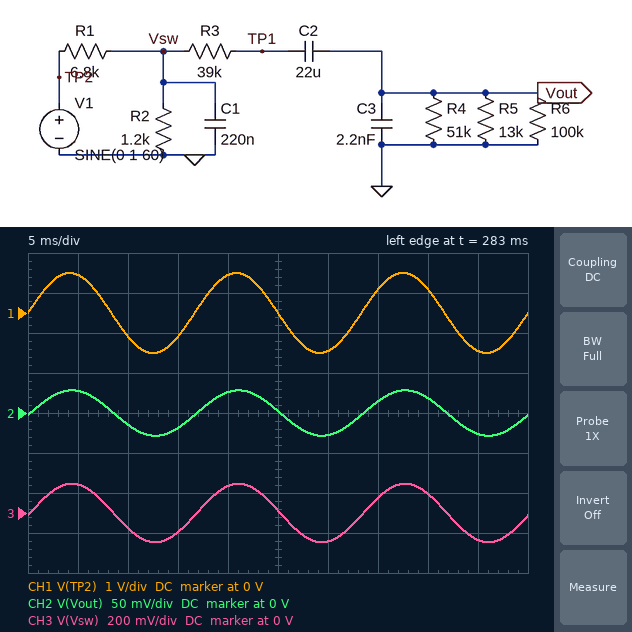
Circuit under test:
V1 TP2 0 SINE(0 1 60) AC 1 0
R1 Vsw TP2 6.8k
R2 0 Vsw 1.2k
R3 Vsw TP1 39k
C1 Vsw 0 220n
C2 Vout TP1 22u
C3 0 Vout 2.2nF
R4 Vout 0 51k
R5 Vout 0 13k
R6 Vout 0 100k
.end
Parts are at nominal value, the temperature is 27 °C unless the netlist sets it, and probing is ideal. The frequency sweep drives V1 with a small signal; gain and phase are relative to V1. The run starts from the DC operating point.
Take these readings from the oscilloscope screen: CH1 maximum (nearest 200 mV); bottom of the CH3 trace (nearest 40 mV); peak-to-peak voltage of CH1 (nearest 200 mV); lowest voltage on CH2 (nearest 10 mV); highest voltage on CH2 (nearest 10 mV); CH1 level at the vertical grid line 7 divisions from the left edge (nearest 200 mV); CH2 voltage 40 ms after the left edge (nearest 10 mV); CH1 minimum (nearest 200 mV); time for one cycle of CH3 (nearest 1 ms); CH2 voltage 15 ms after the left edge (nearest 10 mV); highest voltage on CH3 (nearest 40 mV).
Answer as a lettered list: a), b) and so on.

a) 1.0 V
b) -160 mV
c) 2.0 V
d) -30 mV
e) 30 mV
f) 600 mV
g) 20 mV
h) -1.0 V
i) 17 ms
j) -20 mV
k) 160 mV
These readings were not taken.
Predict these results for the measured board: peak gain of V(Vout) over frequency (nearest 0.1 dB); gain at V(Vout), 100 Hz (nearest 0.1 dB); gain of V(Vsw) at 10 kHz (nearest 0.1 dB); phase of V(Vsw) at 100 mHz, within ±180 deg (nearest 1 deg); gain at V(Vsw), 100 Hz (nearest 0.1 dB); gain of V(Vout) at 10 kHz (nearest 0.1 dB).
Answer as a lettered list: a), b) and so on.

a) -30.9 dB
b) -31.0 dB
c) -39.5 dB
d) -1 deg
e) -16.7 dB
f) -56.9 dB
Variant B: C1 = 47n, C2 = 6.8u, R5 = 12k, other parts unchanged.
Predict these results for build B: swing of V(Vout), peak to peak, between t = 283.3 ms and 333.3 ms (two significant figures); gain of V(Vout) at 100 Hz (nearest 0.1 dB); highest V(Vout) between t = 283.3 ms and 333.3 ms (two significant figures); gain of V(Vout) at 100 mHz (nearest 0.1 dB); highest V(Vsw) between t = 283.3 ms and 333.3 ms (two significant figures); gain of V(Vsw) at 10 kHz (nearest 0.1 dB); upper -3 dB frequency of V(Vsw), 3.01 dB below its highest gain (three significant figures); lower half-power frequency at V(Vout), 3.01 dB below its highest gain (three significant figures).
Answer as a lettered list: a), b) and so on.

a) 54 mV
b) -31.3 dB
c) 27 mV
d) -45.1 dB
e) 150 mV
f) -26.5 dB
g) 3.24 kHz
h) 479 mHz
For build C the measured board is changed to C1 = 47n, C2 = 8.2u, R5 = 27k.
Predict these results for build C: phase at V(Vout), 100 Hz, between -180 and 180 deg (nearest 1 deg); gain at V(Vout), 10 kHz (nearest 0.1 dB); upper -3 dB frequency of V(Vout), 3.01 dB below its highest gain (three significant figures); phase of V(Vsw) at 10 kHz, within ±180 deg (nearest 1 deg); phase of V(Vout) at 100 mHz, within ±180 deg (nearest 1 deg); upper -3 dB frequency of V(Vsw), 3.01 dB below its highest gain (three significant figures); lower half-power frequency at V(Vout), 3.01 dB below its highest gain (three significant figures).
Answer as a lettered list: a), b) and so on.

a) -2 deg
b) -42.8 dB
c) 2.81 kHz
d) -71 deg
e) 74 deg
f) 3.24 kHz
g) 353 mHz
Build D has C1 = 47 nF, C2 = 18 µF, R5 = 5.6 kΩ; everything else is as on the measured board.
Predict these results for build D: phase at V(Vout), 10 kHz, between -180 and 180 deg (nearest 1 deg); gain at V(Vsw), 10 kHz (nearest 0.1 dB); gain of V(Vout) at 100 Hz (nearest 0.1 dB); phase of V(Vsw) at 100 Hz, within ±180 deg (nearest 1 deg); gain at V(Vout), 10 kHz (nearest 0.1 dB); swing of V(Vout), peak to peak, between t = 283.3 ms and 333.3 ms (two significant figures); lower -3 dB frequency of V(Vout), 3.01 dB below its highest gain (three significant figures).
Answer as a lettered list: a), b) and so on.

a) -102 deg
b) -26.5 dB
c) -35.9 dB
d) -2 deg
e) -47.0 dB
f) 32 mV
g) 197 mHz
